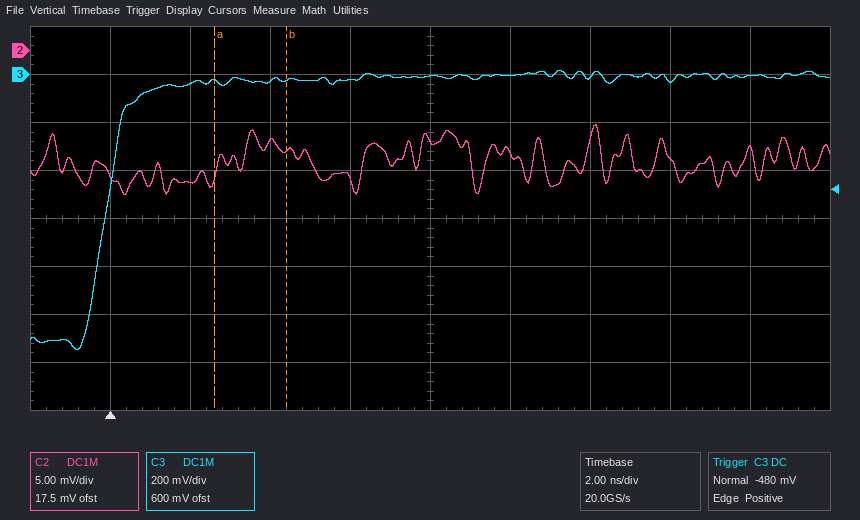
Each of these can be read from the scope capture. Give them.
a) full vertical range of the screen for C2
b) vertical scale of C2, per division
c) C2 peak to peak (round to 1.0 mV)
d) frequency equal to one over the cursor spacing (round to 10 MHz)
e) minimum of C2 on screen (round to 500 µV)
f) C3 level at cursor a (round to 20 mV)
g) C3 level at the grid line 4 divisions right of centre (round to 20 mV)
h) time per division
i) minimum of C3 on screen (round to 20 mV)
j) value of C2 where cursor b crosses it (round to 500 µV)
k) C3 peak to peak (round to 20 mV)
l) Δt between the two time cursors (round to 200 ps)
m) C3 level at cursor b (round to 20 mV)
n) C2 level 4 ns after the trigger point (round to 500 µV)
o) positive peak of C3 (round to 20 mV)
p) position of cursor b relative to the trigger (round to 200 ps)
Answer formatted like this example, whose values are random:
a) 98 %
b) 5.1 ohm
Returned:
a) 40 mV
b) 5 mV
c) 7.0 mV
d) 560 MHz
e) -15.0 mV
f) -20 mV
g) 0 mV
h) 2 ns
i) -1.14 V
j) -10.5 mV
k) 1.16 V
l) 1.8 ns
m) -20 mV
n) -9.5 mV
o) 20 mV
p) +4.4 ns
